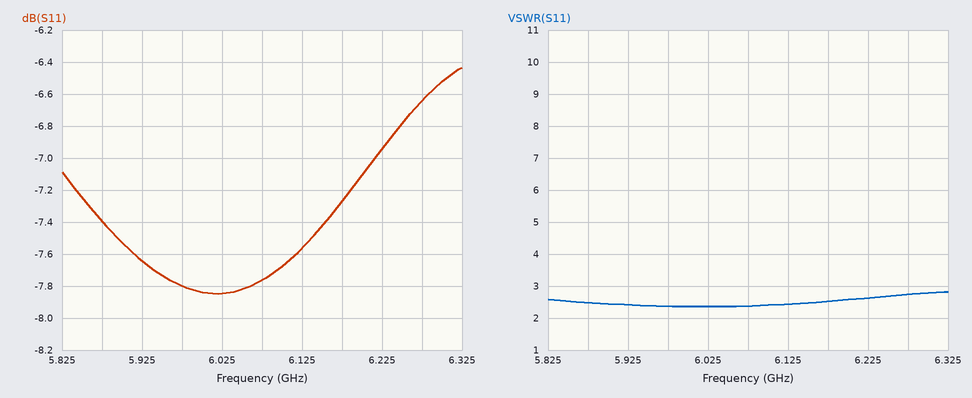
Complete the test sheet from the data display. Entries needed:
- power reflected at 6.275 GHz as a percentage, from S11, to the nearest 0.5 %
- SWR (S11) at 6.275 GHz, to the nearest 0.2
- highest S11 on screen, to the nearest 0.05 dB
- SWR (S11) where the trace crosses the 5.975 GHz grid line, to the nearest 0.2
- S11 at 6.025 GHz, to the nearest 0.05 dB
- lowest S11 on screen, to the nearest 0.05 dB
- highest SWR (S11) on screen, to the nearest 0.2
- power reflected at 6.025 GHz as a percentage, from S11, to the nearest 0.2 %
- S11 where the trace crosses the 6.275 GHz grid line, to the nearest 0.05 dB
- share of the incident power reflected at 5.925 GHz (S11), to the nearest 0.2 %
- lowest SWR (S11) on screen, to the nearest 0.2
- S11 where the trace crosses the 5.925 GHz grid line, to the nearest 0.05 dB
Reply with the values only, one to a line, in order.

21.5 %
2.8
-6.45 dB
2.4
-7.85 dB
-7.85 dB
2.8
16.4 %
-6.65 dB
17.2 %
2.4
-7.65 dB
